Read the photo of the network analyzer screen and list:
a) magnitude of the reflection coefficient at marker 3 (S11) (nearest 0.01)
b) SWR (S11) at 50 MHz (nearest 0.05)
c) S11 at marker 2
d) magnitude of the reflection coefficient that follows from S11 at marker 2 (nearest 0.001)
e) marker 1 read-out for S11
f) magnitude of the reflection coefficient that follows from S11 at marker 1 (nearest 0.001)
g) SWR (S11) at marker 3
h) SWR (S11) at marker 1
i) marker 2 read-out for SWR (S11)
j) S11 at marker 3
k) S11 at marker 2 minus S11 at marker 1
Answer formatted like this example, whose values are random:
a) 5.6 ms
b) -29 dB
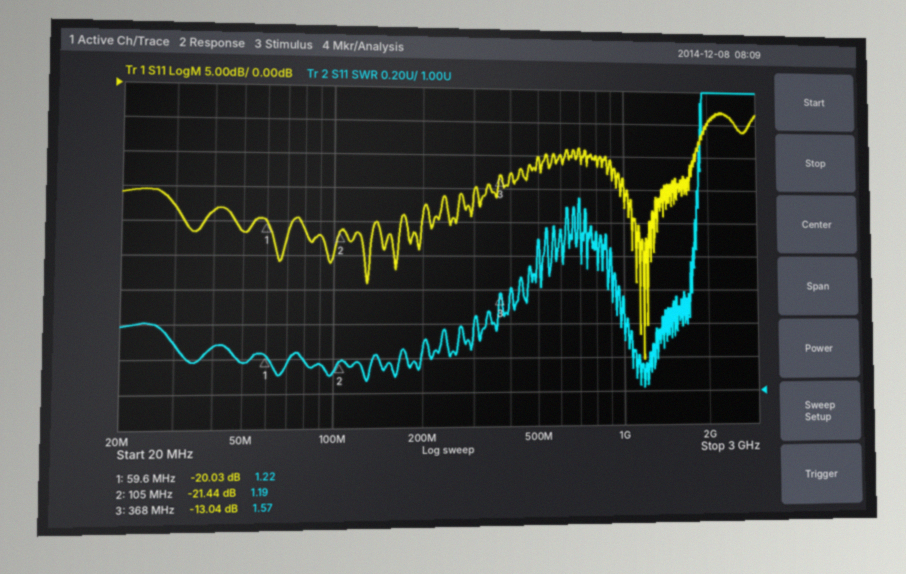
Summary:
a) 0.22
b) 1.20
c) -21.44 dB
d) 0.085
e) -20.03 dB
f) 0.100
g) 1.57
h) 1.22
i) 1.19
j) -13.04 dB
k) -1.41 dB
